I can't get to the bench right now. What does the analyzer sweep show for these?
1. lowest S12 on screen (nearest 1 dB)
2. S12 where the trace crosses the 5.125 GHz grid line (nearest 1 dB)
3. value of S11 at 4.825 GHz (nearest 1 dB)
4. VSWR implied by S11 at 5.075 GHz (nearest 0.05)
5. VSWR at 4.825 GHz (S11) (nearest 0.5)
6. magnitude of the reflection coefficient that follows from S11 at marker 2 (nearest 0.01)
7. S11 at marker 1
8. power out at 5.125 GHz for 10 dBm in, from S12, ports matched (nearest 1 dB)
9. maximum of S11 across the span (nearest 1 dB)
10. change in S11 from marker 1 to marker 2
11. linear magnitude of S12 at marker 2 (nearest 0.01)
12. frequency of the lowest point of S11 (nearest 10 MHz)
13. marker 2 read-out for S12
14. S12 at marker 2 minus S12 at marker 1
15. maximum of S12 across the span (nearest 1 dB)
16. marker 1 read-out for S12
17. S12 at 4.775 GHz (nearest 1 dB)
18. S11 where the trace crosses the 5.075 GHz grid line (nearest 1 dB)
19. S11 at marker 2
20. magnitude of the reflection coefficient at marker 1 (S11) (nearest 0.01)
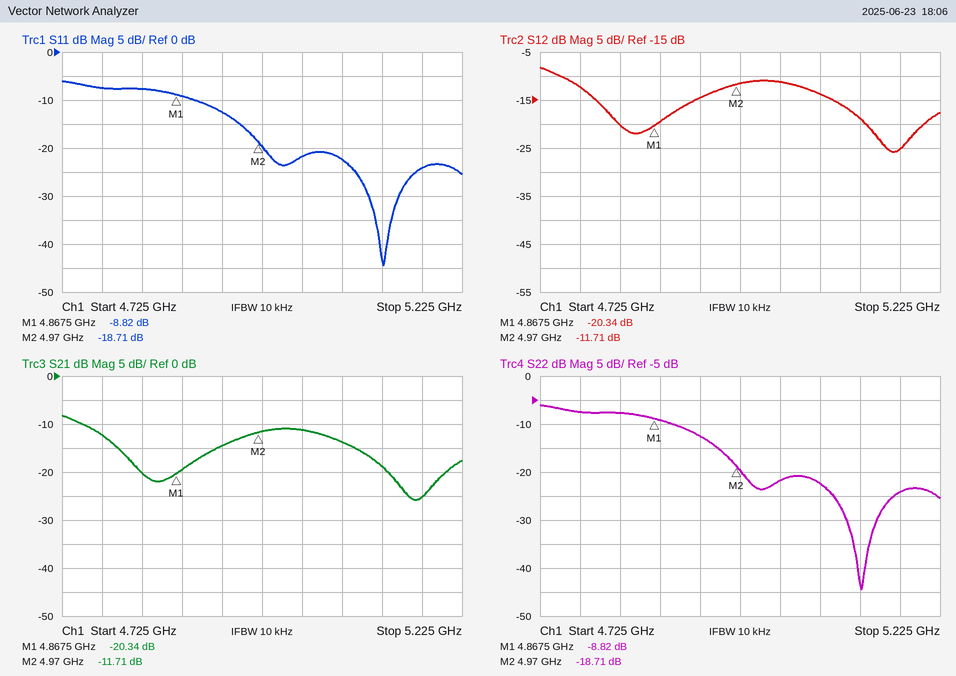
-26 dB
-19 dB
-8 dB
1.15
2.5
0.12
-8.82 dB
-9 dBm
-6 dB
-9.89 dB
0.26
5.13 GHz
-11.71 dB
8.63 dB
-8 dB
-20.34 dB
-12 dB
-22 dB
-18.71 dB
0.36
